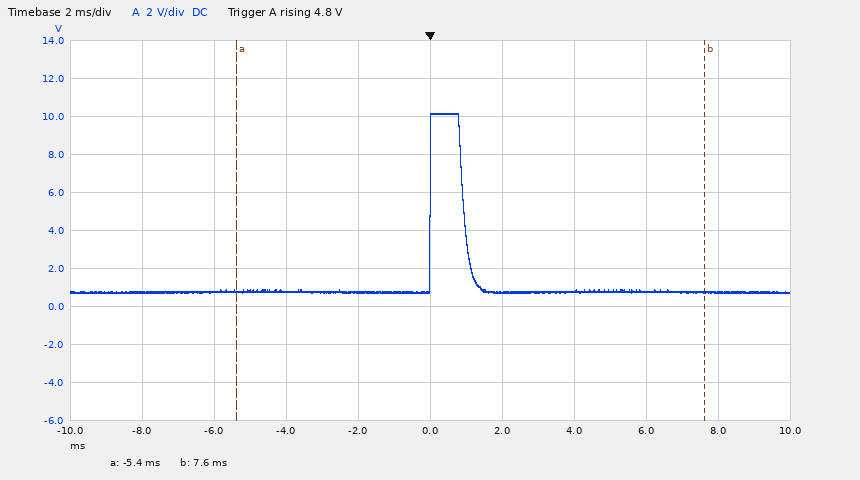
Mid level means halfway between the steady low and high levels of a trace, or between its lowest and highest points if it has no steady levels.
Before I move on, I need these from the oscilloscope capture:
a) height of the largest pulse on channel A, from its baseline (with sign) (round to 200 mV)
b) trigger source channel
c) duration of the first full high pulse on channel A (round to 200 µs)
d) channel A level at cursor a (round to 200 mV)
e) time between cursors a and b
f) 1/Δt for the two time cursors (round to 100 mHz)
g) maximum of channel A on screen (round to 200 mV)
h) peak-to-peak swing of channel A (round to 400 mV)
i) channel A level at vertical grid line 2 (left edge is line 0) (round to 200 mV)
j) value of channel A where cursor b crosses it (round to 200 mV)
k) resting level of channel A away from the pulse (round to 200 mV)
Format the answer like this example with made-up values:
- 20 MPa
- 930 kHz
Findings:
- +9.4 V
- channel A
- 1.0 ms
- 800 mV
- 13.0 ms
- 76.9 Hz
- 10.2 V
- 9.6 V
- 800 mV
- 800 mV
- 800 mV
